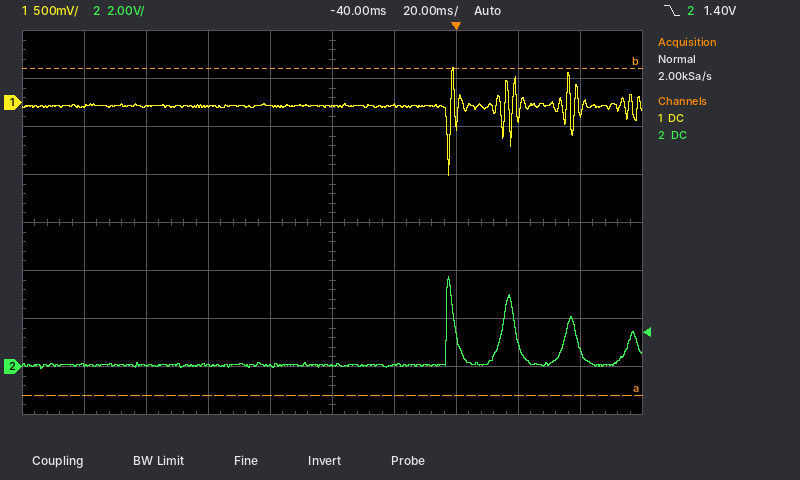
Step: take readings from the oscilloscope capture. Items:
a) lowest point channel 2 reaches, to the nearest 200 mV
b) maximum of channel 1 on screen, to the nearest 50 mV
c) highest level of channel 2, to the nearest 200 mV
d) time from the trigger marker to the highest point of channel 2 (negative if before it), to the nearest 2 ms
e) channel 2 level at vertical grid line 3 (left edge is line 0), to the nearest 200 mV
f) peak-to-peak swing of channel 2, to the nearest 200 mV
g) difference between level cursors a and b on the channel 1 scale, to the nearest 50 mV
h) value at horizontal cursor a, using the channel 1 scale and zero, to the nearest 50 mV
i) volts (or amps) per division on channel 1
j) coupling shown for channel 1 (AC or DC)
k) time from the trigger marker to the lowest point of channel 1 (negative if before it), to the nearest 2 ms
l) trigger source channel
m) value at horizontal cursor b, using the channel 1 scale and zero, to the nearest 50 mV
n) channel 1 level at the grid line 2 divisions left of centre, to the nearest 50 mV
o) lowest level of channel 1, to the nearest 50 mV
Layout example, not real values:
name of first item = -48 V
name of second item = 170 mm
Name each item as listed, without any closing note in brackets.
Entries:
lowest point channel 2 reaches, to the nearest 200 mV = 0.0 V
maximum of channel 1 on screen, to the nearest 50 mV = 350 mV
highest level of channel 2, to the nearest 200 mV = 3.8 V
time from the trigger marker to the highest point of channel 2 (negative if before it), to the nearest 2 ms = -2 ms
channel 2 level at vertical grid line 3 (left edge is line 0), to the nearest 200 mV = 0.0 V
peak-to-peak swing of channel 2, to the nearest 200 mV = 3.8 V
difference between level cursors a and b on the channel 1 scale, to the nearest 50 mV = 3.40 V
value at horizontal cursor a, using the channel 1 scale and zero, to the nearest 50 mV = -3.05 V
volts (or amps) per division on channel 1 = 500 mV
coupling shown for channel 1 = DC
time from the trigger marker to the lowest point of channel 1 (negative if before it), to the nearest 2 ms = -2 ms
trigger source channel = channel 2
value at horizontal cursor b, using the channel 1 scale and zero, to the nearest 50 mV = 350 mV
channel 1 level at the grid line 2 divisions left of centre, to the nearest 50 mV = -50 mV
lowest level of channel 1, to the nearest 50 mV = -750 mV
